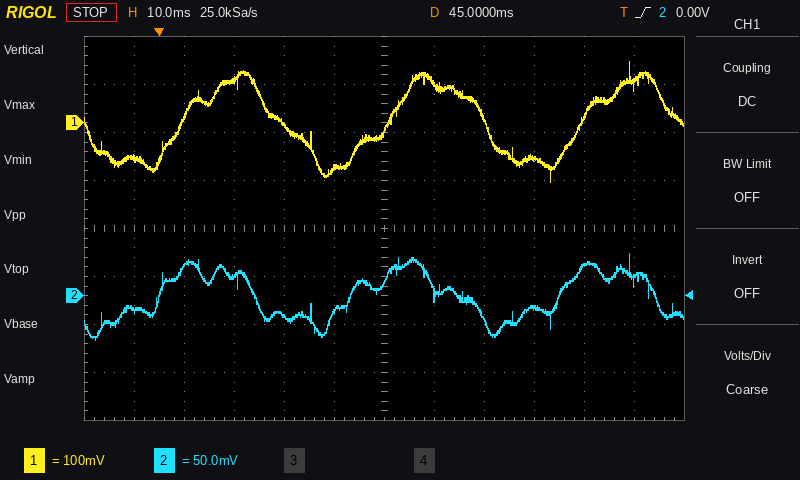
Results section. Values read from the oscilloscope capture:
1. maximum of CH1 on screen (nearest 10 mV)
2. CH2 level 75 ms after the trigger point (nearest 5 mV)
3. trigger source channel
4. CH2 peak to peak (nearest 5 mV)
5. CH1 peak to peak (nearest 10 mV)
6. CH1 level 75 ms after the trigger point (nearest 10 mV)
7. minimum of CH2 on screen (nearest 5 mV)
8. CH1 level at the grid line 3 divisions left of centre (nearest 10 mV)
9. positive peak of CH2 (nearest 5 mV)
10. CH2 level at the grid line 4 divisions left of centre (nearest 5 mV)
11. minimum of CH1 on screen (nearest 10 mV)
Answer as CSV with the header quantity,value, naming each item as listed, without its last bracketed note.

quantity,value
maximum of CH1 on screen,130 mV
CH2 level 75 ms after the trigger point,-10 mV
trigger source channel,CH2
CH2 peak to peak,90 mV
CH1 peak to peak,250 mV
CH1 level 75 ms after the trigger point,-70 mV
minimum of CH2 on screen,-45 mV
CH1 level at the grid line 3 divisions left of centre,90 mV
positive peak of CH2,45 mV
CH2 level at the grid line 4 divisions left of centre,30 mV
minimum of CH1 on screen,-120 mV
